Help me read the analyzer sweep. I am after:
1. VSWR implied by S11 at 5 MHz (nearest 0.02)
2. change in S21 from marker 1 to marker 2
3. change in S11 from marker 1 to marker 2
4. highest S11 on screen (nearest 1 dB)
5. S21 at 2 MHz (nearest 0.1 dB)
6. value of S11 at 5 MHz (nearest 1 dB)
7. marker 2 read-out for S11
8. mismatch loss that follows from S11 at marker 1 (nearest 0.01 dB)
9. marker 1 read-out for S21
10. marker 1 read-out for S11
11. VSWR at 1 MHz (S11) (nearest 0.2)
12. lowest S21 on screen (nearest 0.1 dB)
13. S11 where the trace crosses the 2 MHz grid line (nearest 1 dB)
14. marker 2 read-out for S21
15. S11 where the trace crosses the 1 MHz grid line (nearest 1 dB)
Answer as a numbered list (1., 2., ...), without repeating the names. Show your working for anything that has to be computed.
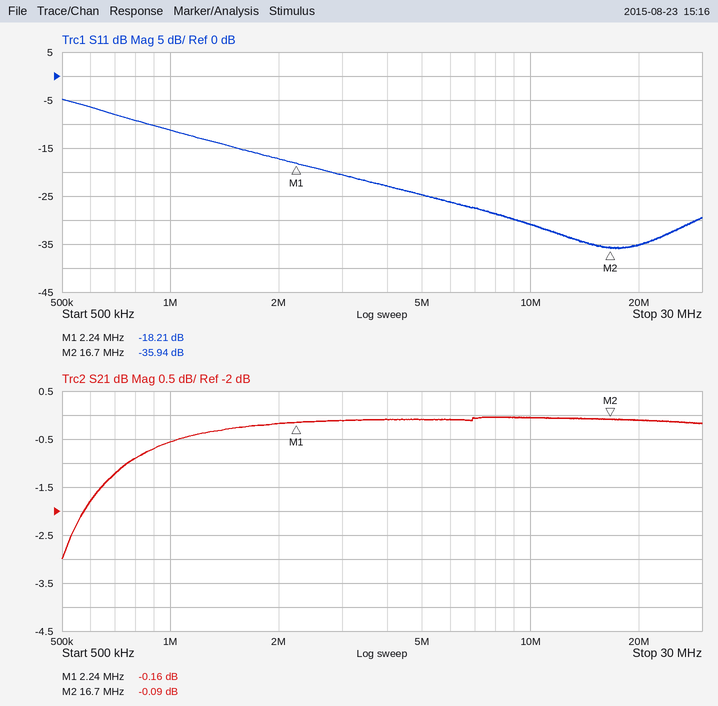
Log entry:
1. |Γ| = 10^(-25/20) = 0.0562; VSWR = (1 + 0.0562)/(1 − 0.0562) ≈ 1.12
2. -0.09 − (-0.16) = 0.07 dB
3. -35.94 − (-18.21) = -17.73 dB
4. -5 dB
5. -0.2 dB
6. -25 dB
7. -35.94 dB
8. −10 log10(1 − 10^(-18.21/10)) ≈ 0.07 dB
9. -0.16 dB
10. -18.21 dB
11. |Γ| = 10^(-11/20) = 0.2818; VSWR = (1 + 0.2818)/(1 − 0.2818) ≈ 1.8
12. -3.0 dB
13. -17 dB
14. -0.09 dB
15. -11 dB
